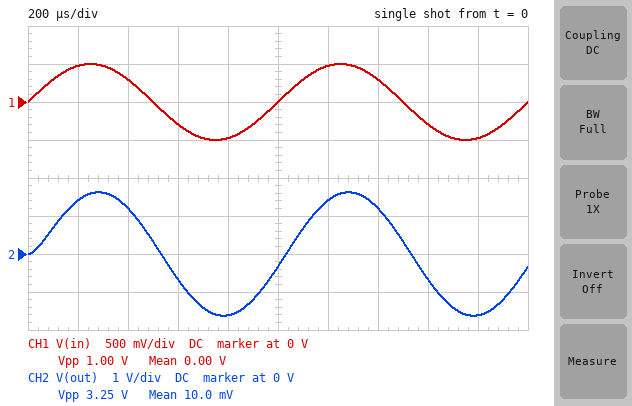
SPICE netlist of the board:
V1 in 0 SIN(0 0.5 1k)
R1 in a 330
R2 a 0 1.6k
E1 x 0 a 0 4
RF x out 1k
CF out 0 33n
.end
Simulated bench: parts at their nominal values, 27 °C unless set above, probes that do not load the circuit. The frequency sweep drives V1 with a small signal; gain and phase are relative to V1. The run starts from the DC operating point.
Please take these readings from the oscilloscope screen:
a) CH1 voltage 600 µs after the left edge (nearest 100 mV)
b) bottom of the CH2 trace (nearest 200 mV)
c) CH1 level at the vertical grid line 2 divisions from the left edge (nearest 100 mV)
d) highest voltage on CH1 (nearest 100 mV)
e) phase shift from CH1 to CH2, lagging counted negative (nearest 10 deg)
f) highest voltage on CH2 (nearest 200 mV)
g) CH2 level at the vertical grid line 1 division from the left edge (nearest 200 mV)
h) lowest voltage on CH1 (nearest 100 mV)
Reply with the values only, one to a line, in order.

-300 mV
-1.6 V
300 mV
500 mV
-10 deg
1.6 V
1.4 V
-500 mV
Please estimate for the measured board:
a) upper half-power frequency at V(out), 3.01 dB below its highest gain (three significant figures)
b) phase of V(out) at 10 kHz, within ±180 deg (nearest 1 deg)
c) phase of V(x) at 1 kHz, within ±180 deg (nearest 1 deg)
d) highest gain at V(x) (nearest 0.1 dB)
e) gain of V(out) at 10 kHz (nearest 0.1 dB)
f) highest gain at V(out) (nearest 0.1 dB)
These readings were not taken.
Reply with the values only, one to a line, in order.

4.82 kHz
-64 deg
0 deg
10.4 dB
3.2 dB
10.4 dB
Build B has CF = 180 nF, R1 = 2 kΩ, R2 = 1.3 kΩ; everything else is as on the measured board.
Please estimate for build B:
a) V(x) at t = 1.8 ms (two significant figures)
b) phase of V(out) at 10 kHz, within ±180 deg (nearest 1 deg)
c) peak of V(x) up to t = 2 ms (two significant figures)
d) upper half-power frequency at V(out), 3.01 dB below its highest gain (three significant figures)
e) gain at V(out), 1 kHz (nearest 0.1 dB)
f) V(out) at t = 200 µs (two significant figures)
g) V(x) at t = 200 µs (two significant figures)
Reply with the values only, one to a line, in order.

-750 mV
-85 deg
790 mV
884 Hz
0.4 dB
340 mV
750 mV
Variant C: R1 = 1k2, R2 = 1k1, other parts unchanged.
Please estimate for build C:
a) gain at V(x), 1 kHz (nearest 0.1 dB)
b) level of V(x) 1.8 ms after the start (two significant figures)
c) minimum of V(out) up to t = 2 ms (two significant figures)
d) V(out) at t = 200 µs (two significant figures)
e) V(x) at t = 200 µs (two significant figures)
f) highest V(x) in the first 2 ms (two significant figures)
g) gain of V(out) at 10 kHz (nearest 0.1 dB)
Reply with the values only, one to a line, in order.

5.6 dB
-910 mV
-940 mV
810 mV
910 mV
960 mV
-1.6 dB
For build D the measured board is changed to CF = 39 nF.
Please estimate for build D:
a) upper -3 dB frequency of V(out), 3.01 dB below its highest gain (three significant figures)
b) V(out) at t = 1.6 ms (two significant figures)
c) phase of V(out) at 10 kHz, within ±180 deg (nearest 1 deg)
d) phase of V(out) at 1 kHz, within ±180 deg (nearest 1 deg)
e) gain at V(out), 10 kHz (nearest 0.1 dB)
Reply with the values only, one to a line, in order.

4.08 kHz
-610 mV
-68 deg
-14 deg
2.0 dB
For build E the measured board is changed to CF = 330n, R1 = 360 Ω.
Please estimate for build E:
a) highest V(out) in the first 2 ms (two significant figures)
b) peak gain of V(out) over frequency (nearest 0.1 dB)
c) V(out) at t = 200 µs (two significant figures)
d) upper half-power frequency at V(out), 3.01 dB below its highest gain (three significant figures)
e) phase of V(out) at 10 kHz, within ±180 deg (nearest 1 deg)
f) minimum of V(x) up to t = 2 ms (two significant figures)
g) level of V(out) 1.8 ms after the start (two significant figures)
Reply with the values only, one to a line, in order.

890 mV
10.3 dB
440 mV
482 Hz
-87 deg
-1.6 V
-490 mV
